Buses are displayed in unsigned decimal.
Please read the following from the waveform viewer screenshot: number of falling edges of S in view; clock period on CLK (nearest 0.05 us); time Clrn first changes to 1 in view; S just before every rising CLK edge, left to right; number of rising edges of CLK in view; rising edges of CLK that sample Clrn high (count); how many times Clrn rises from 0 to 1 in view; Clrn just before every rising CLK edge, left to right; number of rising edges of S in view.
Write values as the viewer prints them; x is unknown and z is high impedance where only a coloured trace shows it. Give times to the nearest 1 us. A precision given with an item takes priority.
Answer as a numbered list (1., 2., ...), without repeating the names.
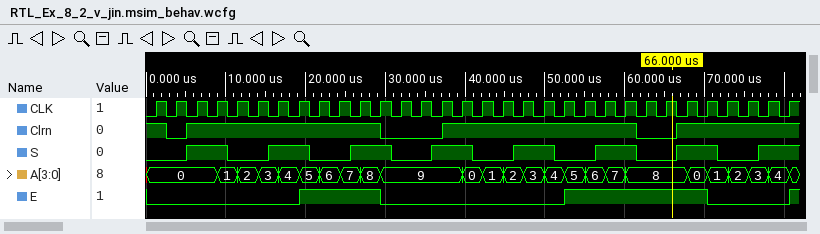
1. 7
2. 2.55 us
3. 5 us
4. 0 0 1 1 0 0 1 1 0 0 1 1 0 0 1 1 0 0 1 1 0 0 1 1 0 0 1 1 0 0 1 1
5. 32
6. 26
7. 3
8. 1 0 1 1 1 1 1 1 1 1 1 1 0 0 0 1 1 1 1 1 1 1 1 1 0 0 1 1 1 1 1 1
9. 8
